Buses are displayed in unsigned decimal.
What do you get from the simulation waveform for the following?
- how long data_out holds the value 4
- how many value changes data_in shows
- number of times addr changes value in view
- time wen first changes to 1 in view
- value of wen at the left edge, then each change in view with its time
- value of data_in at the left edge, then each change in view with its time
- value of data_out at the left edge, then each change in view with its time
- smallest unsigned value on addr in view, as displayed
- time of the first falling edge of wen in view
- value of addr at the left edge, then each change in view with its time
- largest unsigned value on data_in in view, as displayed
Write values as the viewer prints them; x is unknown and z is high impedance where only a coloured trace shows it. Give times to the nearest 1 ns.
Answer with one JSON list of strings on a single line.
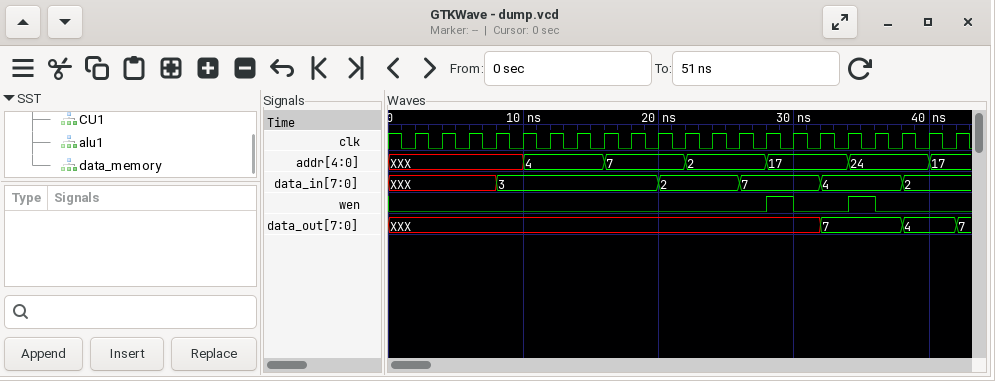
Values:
["4 ns", "5", "6", "28 ns", "0, 1 at 28 ns, 0 at 30 ns, 1 at 34 ns, 0 at 36 ns", "XXX, 3 at 8 ns, 2 at 20 ns, 7 at 26 ns, 4 at 32 ns, 2 at 38 ns", "XXX, 7 at 32 ns, 4 at 38 ns, 7 at 42 ns", "2", "30 ns", "XXX, 4 at 10 ns, 7 at 16 ns, 2 at 22 ns, 17 at 28 ns, 24 at 34 ns, 17 at 40 ns", "7"]
